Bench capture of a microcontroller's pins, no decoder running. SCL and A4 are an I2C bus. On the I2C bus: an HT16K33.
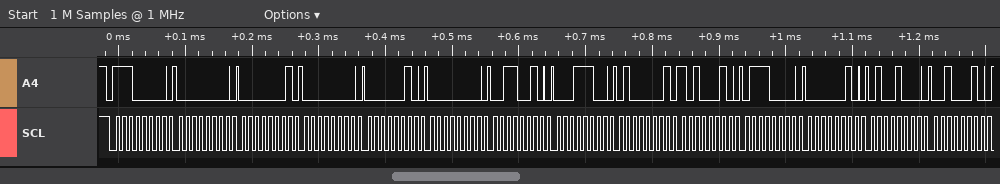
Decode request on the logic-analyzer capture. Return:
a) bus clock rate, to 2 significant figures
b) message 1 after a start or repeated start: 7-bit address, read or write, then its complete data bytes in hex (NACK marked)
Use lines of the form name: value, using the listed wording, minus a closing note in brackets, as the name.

bus clock rate, to 2 significant figures: 100 kHz
message 1 after a start or repeated start: 7-bit address, read or write, then its complete data bytes in hex: 0x70 write: 00 01 00 02 00 32 1C 41 A2 70 02 48 22
